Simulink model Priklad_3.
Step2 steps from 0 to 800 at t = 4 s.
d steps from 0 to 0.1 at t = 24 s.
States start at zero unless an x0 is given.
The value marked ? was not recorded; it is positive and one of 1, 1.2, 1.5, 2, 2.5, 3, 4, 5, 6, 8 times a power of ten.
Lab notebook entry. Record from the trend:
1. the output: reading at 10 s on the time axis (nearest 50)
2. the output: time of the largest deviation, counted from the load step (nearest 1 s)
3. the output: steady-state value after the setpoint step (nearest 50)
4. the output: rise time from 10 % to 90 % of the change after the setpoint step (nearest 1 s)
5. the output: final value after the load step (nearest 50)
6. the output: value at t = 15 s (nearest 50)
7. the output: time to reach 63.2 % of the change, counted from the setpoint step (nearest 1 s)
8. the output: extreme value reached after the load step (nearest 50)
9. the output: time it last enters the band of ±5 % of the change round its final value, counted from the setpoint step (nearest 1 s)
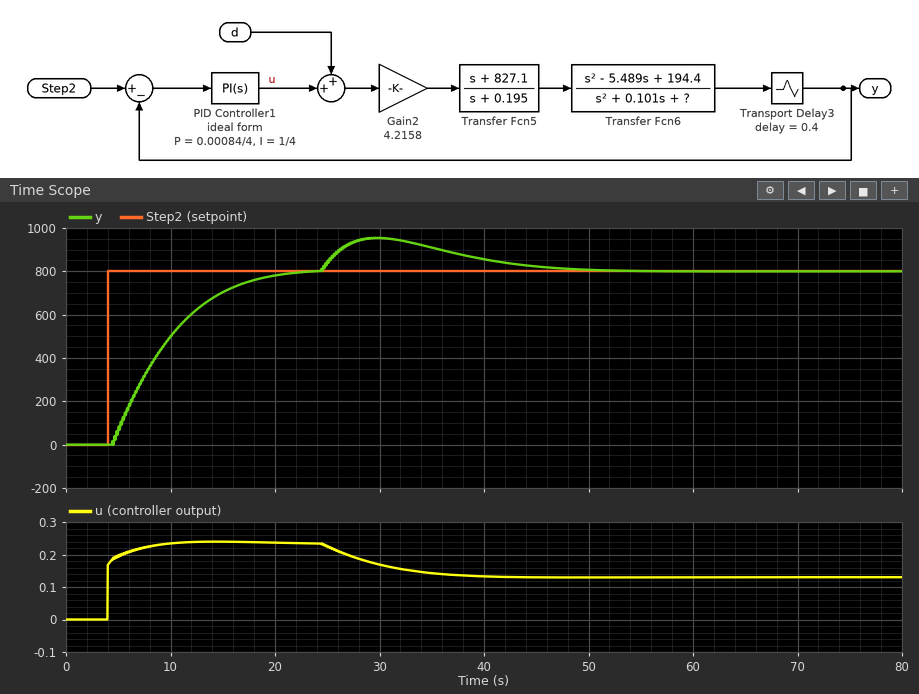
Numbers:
500
6 s
800
11 s
800
700
6 s
950
14 s
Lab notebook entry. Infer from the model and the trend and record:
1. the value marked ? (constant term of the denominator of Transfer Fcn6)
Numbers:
1000
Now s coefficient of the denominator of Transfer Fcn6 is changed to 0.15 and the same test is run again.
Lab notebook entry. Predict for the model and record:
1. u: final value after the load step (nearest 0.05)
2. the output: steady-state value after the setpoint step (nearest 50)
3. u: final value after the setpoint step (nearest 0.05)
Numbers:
0.15
800
0.25
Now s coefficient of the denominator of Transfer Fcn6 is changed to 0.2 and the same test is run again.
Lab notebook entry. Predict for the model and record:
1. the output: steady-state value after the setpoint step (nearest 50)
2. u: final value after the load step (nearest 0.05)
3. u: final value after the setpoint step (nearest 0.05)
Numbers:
800
0.15
0.25
